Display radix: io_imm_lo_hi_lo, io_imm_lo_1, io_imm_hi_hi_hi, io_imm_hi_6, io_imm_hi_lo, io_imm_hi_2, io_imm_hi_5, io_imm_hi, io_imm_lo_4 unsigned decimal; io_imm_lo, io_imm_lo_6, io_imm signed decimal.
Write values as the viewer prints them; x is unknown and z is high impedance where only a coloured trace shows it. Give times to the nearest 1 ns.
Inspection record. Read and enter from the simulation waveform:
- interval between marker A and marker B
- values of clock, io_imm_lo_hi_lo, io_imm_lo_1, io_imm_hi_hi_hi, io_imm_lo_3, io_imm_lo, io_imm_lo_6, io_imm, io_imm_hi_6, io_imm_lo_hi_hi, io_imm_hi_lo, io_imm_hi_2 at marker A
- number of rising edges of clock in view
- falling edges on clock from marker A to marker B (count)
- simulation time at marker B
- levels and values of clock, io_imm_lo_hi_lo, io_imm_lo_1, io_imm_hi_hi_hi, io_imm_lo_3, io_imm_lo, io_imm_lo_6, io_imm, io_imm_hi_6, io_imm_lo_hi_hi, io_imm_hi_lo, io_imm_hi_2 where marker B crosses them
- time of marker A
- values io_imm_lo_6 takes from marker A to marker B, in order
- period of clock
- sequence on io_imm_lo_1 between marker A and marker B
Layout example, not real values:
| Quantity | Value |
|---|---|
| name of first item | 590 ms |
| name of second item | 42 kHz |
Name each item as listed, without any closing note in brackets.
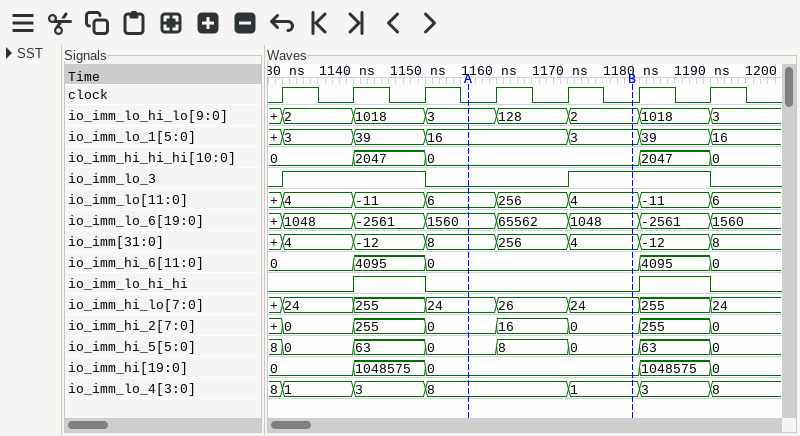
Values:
| Quantity | Value |
|---|---|
| interval between marker A and marker B | 23 ns |
| values of clock, io_imm_lo_hi_lo, io_imm_lo_1, io_imm_hi_hi_hi, io_imm_lo_3, io_imm_lo, io_imm_lo_6, io_imm, io_imm_hi_6, io_imm_lo_hi_hi, io_imm_hi_lo, io_imm_hi_2 at marker A | clock=0, io_imm_lo_hi_lo=3, io_imm_lo_1=16, io_imm_hi_hi_hi=0, io_imm_lo_3=0, io_imm_lo=6, io_imm_lo_6=1560, io_imm=8, io_imm_hi_6=0, io_imm_lo_hi_hi=0, io_imm_hi_lo=24, io_imm_hi_2=0 |
| number of rising edges of clock in view | 7 |
| falling edges on clock from marker A to marker B | 2 |
| simulation time at marker B | 1180 ns |
| levels and values of clock, io_imm_lo_hi_lo, io_imm_lo_1, io_imm_hi_hi_hi, io_imm_lo_3, io_imm_lo, io_imm_lo_6, io_imm, io_imm_hi_6, io_imm_lo_hi_hi, io_imm_hi_lo, io_imm_hi_2 where marker B crosses them | clock=0, io_imm_lo_hi_lo=2, io_imm_lo_1=3, io_imm_hi_hi_hi=0, io_imm_lo_3=1, io_imm_lo=4, io_imm_lo_6=1048, io_imm=4, io_imm_hi_6=0, io_imm_lo_hi_hi=0, io_imm_hi_lo=24, io_imm_hi_2=0 |
| time of marker A | 1157 ns |
| values io_imm_lo_6 takes from marker A to marker B, in order | 1560, 65562, 1048 |
| period of clock | 10 ns |
| sequence on io_imm_lo_1 between marker A and marker B | 16, 3 |
